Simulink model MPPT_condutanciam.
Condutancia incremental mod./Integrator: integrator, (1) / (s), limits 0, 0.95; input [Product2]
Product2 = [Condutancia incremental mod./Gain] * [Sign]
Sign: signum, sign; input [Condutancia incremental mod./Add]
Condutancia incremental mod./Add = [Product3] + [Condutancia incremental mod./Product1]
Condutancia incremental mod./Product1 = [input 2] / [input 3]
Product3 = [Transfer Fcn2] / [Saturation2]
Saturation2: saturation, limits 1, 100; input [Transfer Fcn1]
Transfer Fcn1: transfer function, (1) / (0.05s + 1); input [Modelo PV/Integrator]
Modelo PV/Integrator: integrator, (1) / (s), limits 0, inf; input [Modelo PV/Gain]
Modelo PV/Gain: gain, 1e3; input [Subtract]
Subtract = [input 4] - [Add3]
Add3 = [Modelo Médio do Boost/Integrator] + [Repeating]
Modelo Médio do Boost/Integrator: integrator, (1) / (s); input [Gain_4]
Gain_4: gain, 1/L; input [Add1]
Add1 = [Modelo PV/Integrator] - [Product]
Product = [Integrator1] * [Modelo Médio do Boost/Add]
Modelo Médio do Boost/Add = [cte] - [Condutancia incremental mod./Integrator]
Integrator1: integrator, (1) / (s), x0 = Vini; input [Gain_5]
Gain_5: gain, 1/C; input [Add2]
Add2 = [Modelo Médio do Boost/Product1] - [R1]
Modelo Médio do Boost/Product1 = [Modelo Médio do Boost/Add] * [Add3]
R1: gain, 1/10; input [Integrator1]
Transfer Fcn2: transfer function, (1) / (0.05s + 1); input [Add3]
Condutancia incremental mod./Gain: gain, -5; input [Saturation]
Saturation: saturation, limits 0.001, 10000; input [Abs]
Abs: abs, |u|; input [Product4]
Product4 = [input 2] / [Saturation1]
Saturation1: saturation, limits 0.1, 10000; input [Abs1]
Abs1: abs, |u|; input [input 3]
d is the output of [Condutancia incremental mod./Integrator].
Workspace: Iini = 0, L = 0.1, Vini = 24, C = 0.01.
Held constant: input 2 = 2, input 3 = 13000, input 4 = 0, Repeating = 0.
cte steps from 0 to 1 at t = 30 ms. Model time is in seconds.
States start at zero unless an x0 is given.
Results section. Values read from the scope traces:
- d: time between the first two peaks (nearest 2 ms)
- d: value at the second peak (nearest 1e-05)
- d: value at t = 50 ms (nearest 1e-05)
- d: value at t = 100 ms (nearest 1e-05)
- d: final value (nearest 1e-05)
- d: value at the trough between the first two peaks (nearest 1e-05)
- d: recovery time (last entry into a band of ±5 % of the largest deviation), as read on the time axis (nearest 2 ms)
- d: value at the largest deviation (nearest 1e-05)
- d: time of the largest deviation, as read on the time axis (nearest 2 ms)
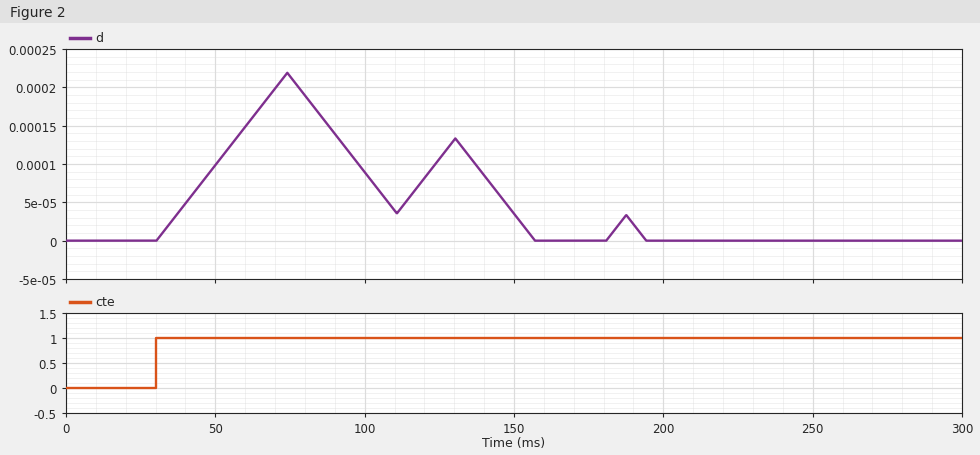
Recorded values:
56 ms
0.00013
0.00010
0.00009
0.00000
0.00004
192 ms
0.00022
74 ms
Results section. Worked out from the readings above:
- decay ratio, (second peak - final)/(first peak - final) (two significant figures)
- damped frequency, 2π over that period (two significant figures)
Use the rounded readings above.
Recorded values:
0.59
0.11 rad/ms
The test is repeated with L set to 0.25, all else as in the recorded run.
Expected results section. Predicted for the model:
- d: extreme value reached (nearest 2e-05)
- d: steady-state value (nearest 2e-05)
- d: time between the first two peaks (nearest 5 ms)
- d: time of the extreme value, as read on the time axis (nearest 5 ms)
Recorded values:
0.00032
0.00000
90 ms
95 ms
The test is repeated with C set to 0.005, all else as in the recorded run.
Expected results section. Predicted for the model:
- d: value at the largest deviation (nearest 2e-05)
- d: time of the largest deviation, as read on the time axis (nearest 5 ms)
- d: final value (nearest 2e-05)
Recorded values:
0.00020
70 ms
0.00000
